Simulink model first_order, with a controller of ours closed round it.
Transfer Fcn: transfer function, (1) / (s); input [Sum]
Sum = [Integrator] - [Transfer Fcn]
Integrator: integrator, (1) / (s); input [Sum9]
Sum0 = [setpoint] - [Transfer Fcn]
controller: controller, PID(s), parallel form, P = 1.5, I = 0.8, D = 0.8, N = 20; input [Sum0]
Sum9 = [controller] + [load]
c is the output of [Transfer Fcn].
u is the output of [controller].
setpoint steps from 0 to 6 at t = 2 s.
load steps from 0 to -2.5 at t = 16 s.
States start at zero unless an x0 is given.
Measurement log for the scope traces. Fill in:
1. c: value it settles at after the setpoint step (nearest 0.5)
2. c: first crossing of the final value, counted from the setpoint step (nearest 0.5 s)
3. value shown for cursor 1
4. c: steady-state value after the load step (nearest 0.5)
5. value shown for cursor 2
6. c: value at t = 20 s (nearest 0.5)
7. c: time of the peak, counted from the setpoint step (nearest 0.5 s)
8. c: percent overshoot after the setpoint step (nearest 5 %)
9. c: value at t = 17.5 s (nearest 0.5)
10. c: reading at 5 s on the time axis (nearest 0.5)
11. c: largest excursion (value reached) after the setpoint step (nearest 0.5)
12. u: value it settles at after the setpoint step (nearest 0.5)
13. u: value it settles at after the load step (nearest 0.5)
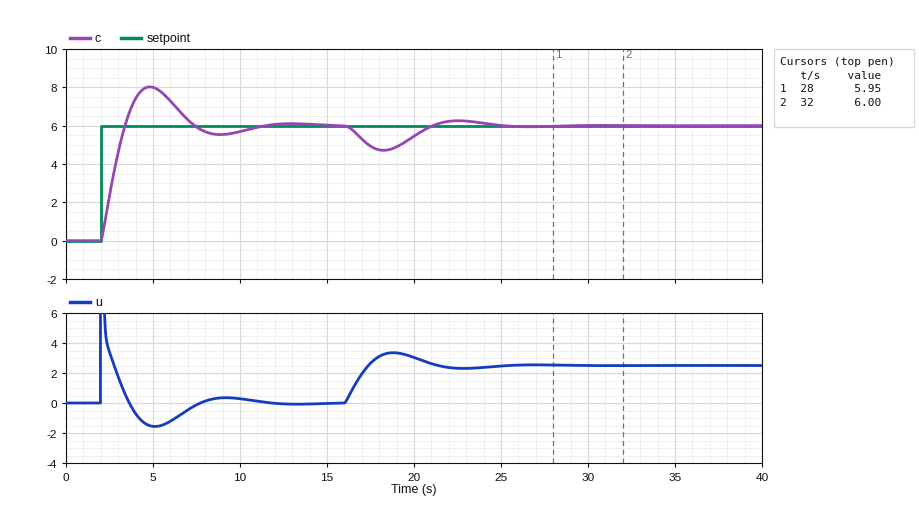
6.0
1.5 s
5.95
6.0
6.00
5.5
3.0 s
35 %
5.0
8.0
8.0
0.0
2.5
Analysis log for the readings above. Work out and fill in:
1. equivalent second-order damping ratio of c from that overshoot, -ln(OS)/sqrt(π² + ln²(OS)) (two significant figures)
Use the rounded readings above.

0.32
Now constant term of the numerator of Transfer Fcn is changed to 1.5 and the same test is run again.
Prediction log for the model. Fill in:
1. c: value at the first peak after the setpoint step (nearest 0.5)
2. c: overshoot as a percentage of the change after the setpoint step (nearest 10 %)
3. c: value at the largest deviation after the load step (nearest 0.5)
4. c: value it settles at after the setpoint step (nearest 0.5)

7.5
20 %
5.0
6.0
